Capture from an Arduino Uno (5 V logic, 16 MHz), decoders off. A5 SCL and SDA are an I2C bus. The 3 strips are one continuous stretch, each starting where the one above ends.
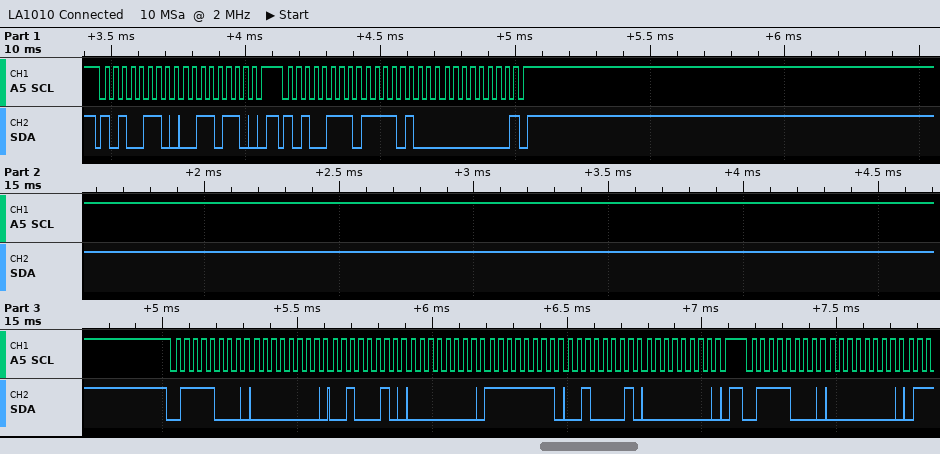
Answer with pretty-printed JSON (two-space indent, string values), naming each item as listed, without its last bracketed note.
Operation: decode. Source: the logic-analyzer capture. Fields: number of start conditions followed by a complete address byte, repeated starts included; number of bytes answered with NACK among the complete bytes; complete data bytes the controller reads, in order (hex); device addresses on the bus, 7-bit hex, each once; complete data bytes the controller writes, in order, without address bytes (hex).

{
  "number of start conditions followed by a complete address byte, repeated starts included": "4",
  "number of bytes answered with NACK among the complete bytes": "1",
  "complete data bytes the controller reads, in order": "F4 00",
  "device addresses on the bus, 7-bit hex, each once": "0x53 0x3C",
  "complete data bytes the controller writes, in order, without address bytes": "36 00 22 00 FF 21 00 00"
}
